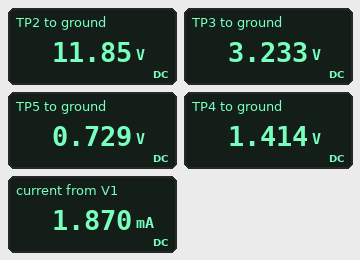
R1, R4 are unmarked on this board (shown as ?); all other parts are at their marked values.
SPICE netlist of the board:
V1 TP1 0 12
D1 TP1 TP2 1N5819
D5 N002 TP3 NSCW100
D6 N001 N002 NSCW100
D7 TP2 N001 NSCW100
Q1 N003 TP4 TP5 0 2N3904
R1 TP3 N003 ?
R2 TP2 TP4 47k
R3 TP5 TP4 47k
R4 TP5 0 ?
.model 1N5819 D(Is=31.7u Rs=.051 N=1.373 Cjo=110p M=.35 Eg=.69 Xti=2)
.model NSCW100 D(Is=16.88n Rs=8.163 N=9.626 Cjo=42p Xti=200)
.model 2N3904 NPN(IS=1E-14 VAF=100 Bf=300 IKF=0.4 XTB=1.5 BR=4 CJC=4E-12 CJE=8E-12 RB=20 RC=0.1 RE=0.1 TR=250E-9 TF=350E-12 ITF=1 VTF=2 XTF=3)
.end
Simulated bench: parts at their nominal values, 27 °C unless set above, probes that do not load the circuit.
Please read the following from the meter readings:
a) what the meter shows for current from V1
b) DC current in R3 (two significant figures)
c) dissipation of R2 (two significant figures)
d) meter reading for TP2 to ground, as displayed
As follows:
1.870 mA
15 µA
2.3 mW
11.85 V
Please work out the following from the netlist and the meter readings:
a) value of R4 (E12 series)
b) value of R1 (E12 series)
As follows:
390 Ω
1.5 kΩ
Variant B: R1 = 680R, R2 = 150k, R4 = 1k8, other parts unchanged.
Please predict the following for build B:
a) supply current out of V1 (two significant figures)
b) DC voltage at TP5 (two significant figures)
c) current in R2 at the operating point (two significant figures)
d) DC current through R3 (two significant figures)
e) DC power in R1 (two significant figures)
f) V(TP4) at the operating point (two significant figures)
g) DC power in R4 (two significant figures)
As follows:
1.4 mA
2.5 V
58 µA
14 µA
1.2 mW
3.1 V
3.4 mW
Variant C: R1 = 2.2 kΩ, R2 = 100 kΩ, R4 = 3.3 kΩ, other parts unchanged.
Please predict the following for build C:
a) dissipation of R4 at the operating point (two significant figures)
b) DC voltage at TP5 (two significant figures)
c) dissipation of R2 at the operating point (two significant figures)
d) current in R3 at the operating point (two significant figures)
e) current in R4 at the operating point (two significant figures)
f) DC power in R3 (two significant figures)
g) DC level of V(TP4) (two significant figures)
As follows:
1.9 mW
2.5 V
770 µW
14 µA
750 µA
9.2 µW
3.1 V
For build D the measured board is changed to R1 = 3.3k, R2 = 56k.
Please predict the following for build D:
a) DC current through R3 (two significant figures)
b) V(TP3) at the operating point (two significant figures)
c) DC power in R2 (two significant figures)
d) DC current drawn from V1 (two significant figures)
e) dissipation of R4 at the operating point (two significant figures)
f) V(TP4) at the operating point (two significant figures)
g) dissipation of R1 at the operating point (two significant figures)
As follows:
14 µA
3.7 V
2.1 mW
1.2 mA
520 µW
1.1 V
3.1 mW
